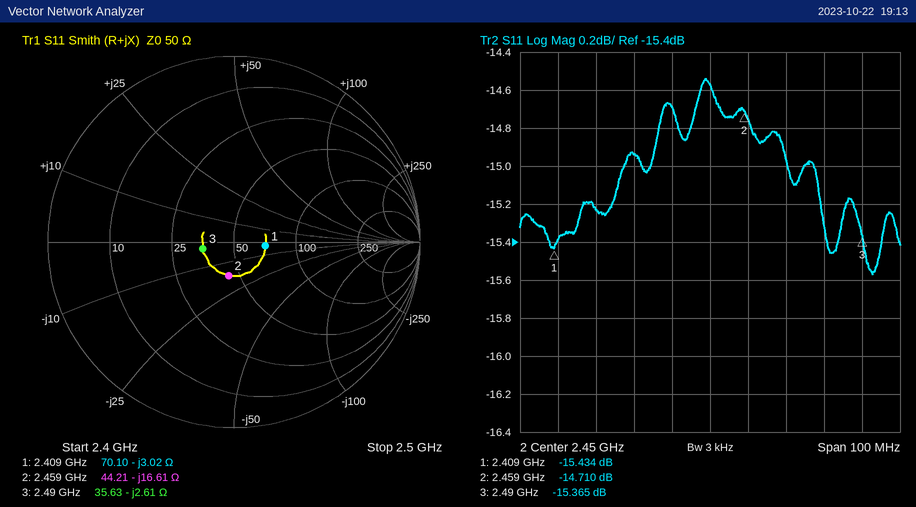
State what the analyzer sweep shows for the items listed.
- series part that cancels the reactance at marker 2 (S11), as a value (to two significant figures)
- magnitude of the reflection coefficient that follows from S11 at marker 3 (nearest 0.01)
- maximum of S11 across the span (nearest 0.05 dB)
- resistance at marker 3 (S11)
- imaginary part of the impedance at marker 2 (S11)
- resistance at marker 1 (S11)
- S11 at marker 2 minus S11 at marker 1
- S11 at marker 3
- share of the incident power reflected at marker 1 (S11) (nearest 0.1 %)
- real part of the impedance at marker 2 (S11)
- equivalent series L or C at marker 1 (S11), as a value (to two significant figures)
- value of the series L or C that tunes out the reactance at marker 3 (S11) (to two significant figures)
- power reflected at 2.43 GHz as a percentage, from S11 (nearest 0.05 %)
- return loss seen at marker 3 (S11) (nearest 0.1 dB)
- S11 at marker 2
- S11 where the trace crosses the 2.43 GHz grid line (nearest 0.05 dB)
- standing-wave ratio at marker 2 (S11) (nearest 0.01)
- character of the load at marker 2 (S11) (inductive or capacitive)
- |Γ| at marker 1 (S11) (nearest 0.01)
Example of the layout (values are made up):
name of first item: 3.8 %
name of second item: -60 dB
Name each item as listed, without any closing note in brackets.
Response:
series part that cancels the reactance at marker 2 (S11), as a value: 1.1 nH
magnitude of the reflection coefficient that follows from S11 at marker 3: 0.17
maximum of S11 across the span: -14.55 dB
resistance at marker 3: 35.63 Ω
imaginary part of the impedance at marker 2: -16.61 Ω
resistance at marker 1: 70.10 Ω
S11 at marker 2 minus S11 at marker 1: 0.724 dB
S11 at marker 3: -15.365 dB
share of the incident power reflected at marker 1 (S11): 2.9 %
real part of the impedance at marker 2: 44.21 Ω
equivalent series L or C at marker 1 (S11), as a value: 22 pF
value of the series L or C that tunes out the reactance at marker 3 (S11): 170 pH
power reflected at 2.43 GHz as a percentage, from S11: 3.20 %
return loss seen at marker 3 (S11): 15.4 dB
S11 at marker 2: -14.710 dB
S11 where the trace crosses the 2.43 GHz grid line: -14.95 dB
standing-wave ratio at marker 2 (S11): 1.45
character of the load at marker 2 (S11): capacitive
|Γ| at marker 1 (S11): 0.17
